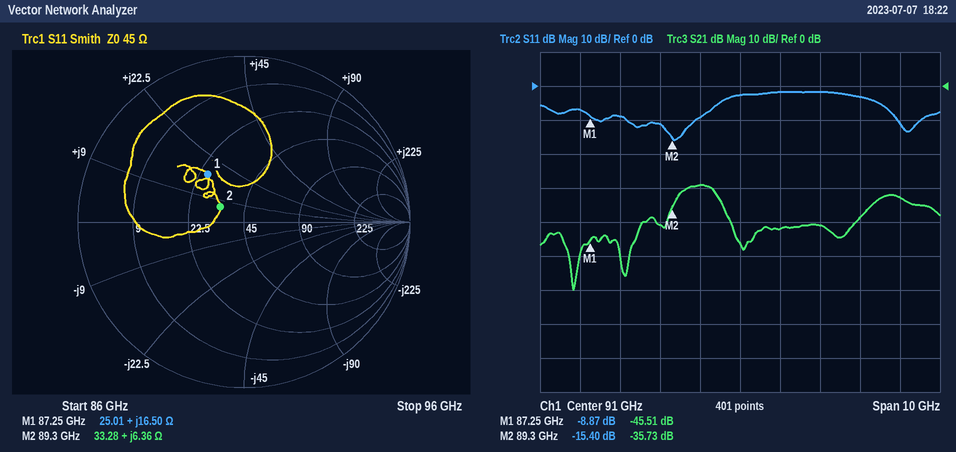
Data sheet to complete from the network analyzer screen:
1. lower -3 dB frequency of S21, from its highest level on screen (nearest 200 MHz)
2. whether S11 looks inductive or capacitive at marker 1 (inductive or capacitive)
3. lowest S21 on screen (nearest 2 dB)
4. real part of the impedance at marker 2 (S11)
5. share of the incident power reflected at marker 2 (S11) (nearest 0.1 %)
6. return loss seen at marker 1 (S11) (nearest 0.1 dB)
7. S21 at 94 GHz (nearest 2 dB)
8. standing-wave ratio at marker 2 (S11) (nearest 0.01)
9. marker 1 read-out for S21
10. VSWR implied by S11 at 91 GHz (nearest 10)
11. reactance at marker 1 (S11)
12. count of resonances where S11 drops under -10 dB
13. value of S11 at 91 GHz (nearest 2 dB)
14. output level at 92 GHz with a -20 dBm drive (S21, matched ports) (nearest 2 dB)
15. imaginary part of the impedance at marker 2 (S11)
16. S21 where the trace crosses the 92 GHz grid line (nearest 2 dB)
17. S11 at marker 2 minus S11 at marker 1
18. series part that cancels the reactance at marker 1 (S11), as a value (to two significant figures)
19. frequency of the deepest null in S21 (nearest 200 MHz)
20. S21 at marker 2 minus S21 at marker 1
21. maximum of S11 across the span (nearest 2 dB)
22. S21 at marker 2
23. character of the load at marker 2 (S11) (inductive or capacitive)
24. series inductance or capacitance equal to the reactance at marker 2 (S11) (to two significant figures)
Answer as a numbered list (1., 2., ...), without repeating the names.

1. 89.4 GHz
2. inductive
3. -60 dB
4. 33.28 Ω
5. 2.9 %
6. 8.9 dB
7. -38 dB
8. 1.41
9. -45.51 dB
10. 10
11. +16.50 Ω
12. 2
13. -2 dB
14. -62 dBm
15. +6.36 Ω
16. -42 dB
17. -6.53 dB
18. 110 fF
19. 86.8 GHz
20. 9.78 dB
21. -2 dB
22. -35.73 dB
23. inductive
24. 11 pH
